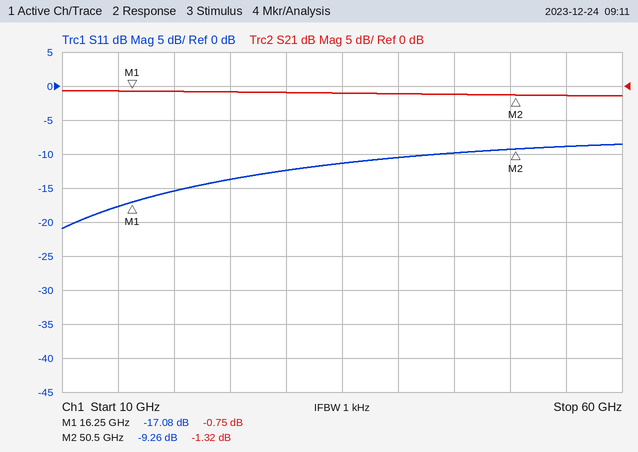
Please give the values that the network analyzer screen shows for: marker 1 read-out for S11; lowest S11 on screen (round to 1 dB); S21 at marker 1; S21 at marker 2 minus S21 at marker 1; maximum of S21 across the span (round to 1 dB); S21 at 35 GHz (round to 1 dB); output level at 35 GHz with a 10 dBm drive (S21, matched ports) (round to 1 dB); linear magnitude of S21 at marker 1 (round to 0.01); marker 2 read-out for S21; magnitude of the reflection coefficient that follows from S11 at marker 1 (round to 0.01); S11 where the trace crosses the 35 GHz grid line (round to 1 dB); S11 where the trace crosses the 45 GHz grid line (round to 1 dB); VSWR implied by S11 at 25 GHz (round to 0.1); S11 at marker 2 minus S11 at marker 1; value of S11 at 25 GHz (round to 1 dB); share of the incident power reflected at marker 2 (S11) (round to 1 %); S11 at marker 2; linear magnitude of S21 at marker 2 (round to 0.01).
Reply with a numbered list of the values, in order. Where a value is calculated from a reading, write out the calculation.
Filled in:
1. -17.08 dB
2. -21 dB
3. -0.75 dB
4. -1.32 − (-0.75) = -0.57 dB
5. -1 dB
6. -1 dB
7. 10 dBm + (-1 dB) = 9 dBm
8. 10^(-0.75/20) ≈ 0.92
9. -1.32 dB
10. 10^(-17.08/20) ≈ 0.14
11. -11 dB
12. -10 dB
13. |Γ| = 10^(-14/20) = 0.1995; VSWR = (1 + 0.1995)/(1 − 0.1995) ≈ 1.5
14. -9.26 − (-17.08) = 7.82 dB
15. -14 dB
16. 10^(-9.26/10) ≈ 12 %
17. -9.26 dB
18. 10^(-1.32/20) ≈ 0.86
